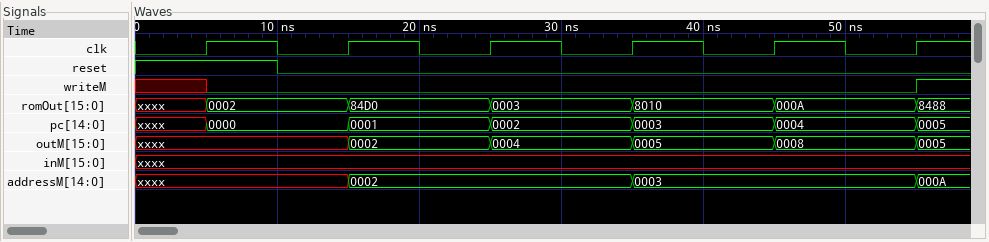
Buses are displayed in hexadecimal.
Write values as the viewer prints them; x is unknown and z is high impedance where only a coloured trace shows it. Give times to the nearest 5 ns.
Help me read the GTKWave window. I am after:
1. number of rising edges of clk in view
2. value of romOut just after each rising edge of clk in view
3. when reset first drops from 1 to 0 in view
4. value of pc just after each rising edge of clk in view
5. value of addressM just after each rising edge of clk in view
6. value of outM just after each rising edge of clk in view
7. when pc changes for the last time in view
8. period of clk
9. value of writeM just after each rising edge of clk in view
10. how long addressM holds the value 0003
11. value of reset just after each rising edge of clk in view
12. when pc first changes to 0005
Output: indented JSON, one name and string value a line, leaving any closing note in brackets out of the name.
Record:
{
  "number of rising edges of clk in view": "6",
  "value of romOut just after each rising edge of clk in view": "0002, 84D0, 0003, 8010, 000A, 8488",
  "when reset first drops from 1 to 0 in view": "10 ns",
  "value of pc just after each rising edge of clk in view": "0000, 0001, 0002, 0003, 0004, 0005",
  "value of addressM just after each rising edge of clk in view": "xxxx, 0002, 0002, 0003, 0003, 000A",
  "value of outM just after each rising edge of clk in view": "xxxx, 0002, 0004, 0005, 0008, 0005",
  "when pc changes for the last time in view": "55 ns",
  "period of clk": "10 ns",
  "value of writeM just after each rising edge of clk in view": "0 0 0 0 0 1",
  "how long addressM holds the value 0003": "20 ns",
  "value of reset just after each rising edge of clk in view": "1 0 0 0 0 0",
  "when pc first changes to 0005": "55 ns"
}
